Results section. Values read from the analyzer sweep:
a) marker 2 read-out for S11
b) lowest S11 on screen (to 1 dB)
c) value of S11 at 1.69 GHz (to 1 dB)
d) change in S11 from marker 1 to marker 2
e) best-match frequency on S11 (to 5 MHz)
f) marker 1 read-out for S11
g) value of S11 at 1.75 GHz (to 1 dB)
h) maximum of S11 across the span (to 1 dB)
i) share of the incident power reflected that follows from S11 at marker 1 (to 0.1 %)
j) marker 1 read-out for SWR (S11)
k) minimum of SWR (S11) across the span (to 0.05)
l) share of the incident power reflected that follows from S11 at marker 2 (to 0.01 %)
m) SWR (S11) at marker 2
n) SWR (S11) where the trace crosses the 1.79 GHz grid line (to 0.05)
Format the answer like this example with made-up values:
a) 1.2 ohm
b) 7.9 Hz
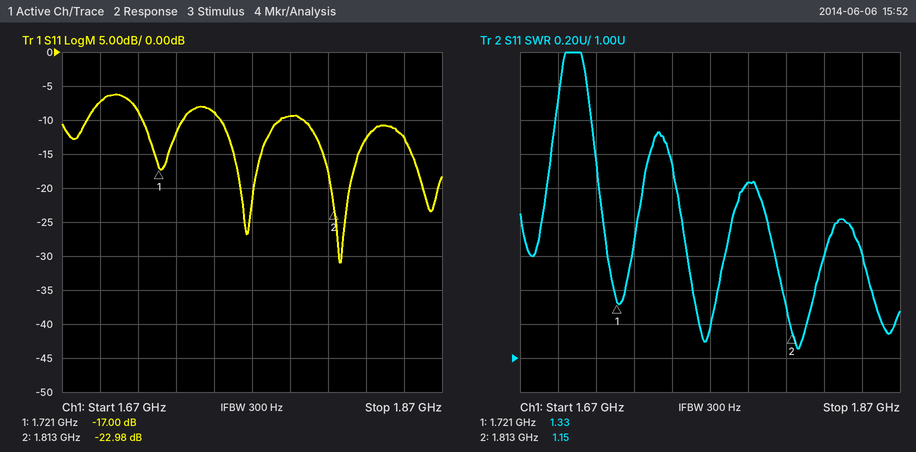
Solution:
a) -22.98 dB
b) -31 dB
c) -7 dB
d) -5.98 dB
e) 1.815 GHz
f) -17.00 dB
g) -9 dB
h) -6 dB
i) 2.0 %
j) 1.33
k) 1.05
l) 0.50 %
m) 1.15
n) 2.05
